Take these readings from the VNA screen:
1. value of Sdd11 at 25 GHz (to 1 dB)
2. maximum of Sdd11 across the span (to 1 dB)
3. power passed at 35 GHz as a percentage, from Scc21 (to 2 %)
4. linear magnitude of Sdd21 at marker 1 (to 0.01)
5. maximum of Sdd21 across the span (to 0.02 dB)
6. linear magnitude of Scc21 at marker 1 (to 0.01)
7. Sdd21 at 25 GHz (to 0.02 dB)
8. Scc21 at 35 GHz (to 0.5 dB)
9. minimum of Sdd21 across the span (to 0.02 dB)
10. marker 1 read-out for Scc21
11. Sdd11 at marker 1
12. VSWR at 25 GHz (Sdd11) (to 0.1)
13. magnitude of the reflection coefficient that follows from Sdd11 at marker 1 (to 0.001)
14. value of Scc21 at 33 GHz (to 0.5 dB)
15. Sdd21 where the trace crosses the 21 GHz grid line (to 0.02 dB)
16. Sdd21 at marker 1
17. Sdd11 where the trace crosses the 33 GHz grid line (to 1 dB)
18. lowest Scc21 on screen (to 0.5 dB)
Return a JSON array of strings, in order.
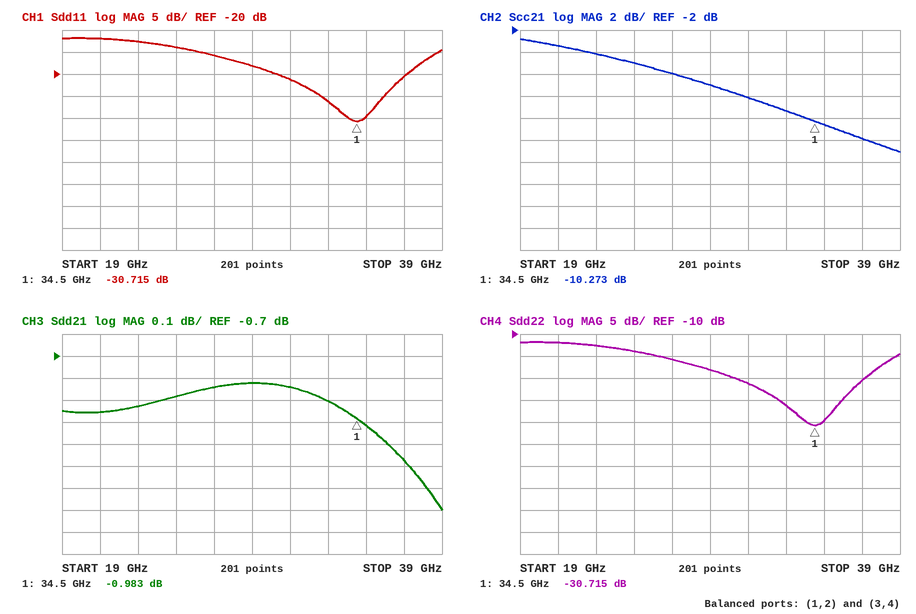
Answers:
["-14 dB", "-12 dB", "8 %", "0.89", "-0.82 dB", "0.31", "-0.88 dB", "-10.5 dB", "-1.40 dB", "-10.273 dB", "-30.715 dB", "1.5", "0.029", "-9.5 dB", "-0.96 dB", "-0.983 dB", "-26 dB", "-13.0 dB"]
